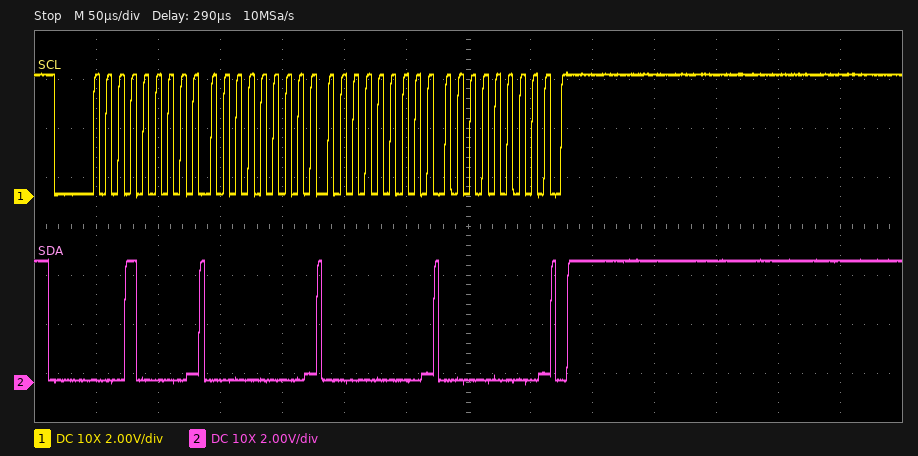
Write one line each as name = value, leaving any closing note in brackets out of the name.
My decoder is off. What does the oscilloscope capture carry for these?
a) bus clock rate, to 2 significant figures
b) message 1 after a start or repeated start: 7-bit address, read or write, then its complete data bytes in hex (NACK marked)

bus clock rate, to 2 significant figures = 100 kHz
message 1 after a start or repeated start: 7-bit address, read or write, then its complete data bytes in hex = 0x08 write: 00 00 00
